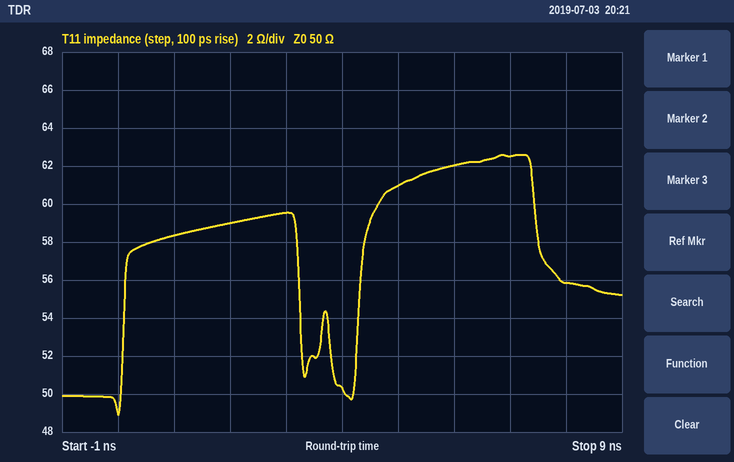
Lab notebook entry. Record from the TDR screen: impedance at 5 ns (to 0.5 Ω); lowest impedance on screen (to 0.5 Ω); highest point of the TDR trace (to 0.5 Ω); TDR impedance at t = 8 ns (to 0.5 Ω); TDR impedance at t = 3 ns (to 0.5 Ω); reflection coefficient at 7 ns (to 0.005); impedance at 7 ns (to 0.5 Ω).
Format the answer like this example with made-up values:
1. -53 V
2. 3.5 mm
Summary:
1. 61.0 Ω
2. 49.0 Ω
3. 62.5 Ω
4. 56.0 Ω
5. 59.5 Ω
6. +0.110
7. 62.5 Ω
